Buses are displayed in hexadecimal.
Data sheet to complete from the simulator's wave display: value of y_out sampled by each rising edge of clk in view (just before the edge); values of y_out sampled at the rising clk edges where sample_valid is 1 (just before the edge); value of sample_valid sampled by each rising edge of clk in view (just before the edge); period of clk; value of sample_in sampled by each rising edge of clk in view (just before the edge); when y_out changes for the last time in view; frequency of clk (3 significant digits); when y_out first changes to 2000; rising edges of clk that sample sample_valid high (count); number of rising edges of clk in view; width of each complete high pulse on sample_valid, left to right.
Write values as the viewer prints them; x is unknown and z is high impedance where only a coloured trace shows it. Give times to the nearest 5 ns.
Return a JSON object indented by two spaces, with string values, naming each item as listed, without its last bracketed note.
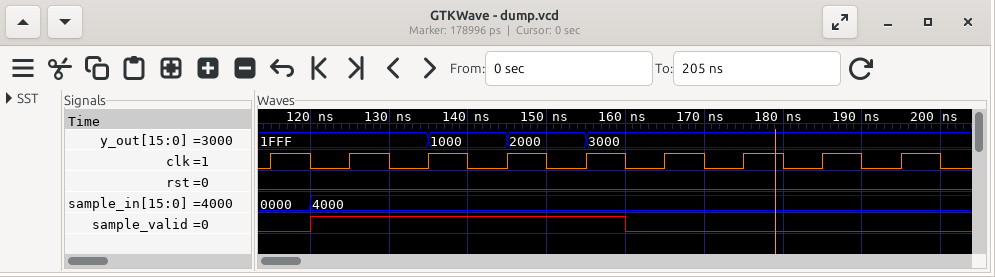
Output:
{
  "value of y_out sampled by each rising edge of clk in view": "1FFF, 1FFF, 1FFF, 1000, 2000, 3000, 3000, 3000, 3000",
  "values of y_out sampled at the rising clk edges where sample_valid is 1": "1FFF, 1FFF, 1000, 2000",
  "value of sample_valid sampled by each rising edge of clk in view": "0 1 1 1 1 0 0 0 0",
  "period of clk": "10 ns",
  "value of sample_in sampled by each rising edge of clk in view": "0000, 4000, 4000, 4000, 4000, 4000, 4000, 4000, 4000",
  "when y_out changes for the last time in view": "155 ns",
  "frequency of clk": "100 MHz",
  "when y_out first changes to 2000": "145 ns",
  "rising edges of clk that sample sample_valid high": "4",
  "number of rising edges of clk in view": "9",
  "width of each complete high pulse on sample_valid, left to right": "40 ns"
}
